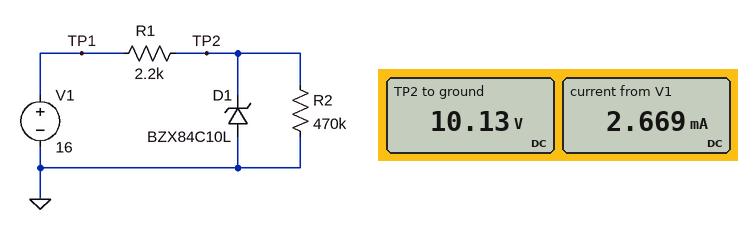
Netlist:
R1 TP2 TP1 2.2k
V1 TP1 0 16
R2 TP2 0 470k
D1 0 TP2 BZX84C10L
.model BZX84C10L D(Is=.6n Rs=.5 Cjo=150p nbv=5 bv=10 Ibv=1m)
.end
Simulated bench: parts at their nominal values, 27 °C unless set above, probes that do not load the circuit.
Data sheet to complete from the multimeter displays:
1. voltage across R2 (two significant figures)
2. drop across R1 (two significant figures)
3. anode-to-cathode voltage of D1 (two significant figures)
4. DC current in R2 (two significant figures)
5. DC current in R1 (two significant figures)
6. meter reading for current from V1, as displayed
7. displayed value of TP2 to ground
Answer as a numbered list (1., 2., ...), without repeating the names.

1. 10 V
2. 5.9 V
3. -10 V
4. 22 µA
5. 2.7 mA
6. 2.669 mA
7. 10.13 V
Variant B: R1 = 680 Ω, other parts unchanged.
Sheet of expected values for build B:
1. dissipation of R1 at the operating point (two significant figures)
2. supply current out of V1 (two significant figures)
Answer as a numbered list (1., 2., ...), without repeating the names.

1. 48 mW
2. 8.4 mA
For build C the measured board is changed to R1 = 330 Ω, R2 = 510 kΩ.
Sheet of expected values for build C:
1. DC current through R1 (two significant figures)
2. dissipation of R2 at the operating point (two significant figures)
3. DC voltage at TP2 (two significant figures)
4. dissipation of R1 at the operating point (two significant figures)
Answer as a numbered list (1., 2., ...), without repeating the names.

1. 17 mA
2. 210 µW
3. 10 V
4. 96 mW
